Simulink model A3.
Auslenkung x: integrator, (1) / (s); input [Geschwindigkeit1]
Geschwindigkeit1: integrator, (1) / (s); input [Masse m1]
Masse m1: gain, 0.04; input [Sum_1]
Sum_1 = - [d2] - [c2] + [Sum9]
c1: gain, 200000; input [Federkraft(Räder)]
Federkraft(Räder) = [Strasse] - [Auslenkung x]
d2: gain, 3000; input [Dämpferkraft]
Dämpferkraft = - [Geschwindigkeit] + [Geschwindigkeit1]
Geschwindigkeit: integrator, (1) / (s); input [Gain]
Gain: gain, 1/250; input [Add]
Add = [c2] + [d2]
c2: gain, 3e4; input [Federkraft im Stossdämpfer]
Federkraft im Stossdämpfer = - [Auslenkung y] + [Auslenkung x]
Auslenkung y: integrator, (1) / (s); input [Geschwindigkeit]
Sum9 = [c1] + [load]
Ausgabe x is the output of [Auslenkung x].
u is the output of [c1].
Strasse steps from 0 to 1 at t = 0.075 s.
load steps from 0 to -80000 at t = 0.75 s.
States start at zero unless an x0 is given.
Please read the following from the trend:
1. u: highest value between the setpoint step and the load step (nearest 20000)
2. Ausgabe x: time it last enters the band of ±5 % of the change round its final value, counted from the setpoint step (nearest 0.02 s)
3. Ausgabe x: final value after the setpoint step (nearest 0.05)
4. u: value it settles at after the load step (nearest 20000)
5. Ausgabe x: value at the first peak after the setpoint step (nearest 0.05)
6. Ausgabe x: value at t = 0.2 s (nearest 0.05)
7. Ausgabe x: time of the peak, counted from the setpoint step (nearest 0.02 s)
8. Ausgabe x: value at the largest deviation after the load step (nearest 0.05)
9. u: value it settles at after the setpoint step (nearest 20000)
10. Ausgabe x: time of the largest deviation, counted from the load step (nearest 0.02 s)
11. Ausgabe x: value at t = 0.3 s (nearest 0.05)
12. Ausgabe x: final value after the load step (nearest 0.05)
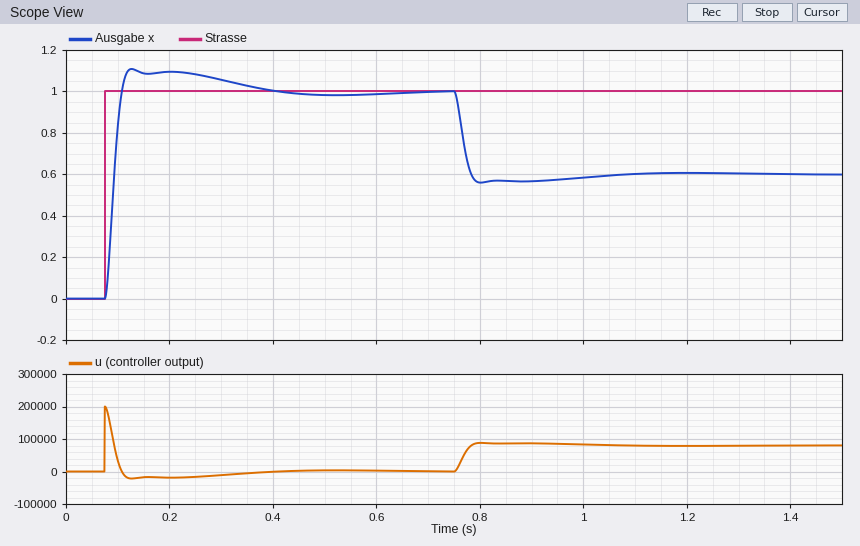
200000
0.24 s
1.00
80000
1.10
1.10
0.06 s
0.55
0
0.06 s
1.05
0.60
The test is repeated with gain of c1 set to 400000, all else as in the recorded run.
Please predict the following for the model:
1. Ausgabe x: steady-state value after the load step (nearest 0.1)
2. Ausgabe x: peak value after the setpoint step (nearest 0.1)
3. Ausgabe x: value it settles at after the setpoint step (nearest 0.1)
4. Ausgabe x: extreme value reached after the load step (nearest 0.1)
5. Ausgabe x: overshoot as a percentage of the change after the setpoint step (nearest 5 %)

0.8
1.2
1.0
0.8
20 %
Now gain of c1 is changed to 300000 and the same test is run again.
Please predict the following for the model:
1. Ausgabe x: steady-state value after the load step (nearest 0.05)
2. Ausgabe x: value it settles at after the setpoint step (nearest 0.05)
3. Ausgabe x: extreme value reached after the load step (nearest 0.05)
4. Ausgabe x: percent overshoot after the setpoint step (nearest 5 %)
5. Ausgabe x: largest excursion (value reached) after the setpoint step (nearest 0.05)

0.75
1.00
0.70
15 %
1.15
